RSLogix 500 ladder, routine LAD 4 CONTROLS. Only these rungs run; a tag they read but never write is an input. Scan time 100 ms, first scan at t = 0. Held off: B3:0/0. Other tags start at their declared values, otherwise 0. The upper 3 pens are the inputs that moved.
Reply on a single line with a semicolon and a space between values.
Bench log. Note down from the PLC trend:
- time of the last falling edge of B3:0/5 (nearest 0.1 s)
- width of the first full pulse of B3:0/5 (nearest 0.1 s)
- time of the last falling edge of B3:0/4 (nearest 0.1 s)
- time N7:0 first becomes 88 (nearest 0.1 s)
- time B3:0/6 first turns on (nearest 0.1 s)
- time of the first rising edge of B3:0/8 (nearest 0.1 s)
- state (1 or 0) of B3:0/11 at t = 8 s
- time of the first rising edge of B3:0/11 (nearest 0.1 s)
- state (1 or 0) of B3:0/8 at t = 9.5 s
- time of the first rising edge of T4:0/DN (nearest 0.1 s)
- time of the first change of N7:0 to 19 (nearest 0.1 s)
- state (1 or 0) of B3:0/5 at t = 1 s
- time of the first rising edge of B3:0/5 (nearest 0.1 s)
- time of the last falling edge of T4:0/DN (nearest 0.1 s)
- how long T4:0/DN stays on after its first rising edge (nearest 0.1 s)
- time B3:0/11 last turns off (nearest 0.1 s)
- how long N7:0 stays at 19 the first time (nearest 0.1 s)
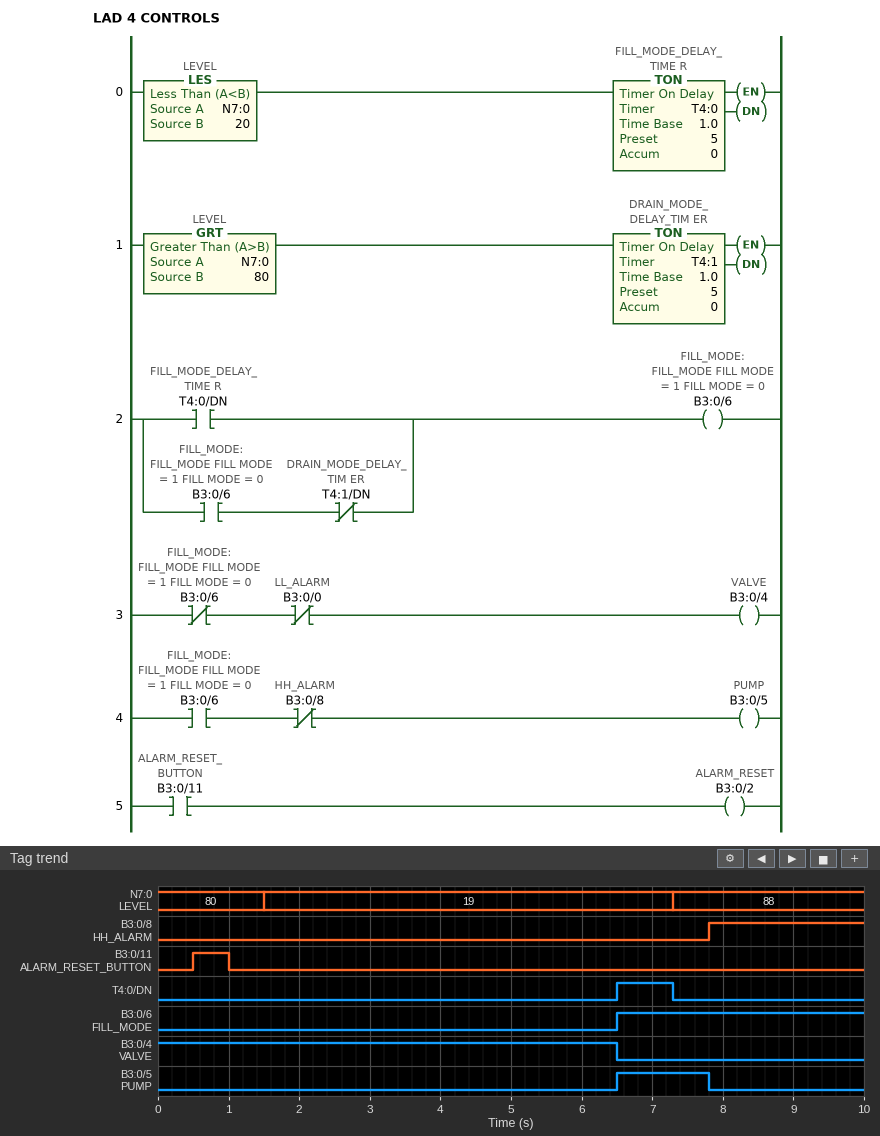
7.8 s; 1.3 s; 6.5 s; 7.3 s; 6.5 s; 7.8 s; 0; 0.5 s; 1; 6.5 s; 1.5 s; 0; 6.5 s; 7.3 s; 0.8 s; 1.0 s; 5.8 s
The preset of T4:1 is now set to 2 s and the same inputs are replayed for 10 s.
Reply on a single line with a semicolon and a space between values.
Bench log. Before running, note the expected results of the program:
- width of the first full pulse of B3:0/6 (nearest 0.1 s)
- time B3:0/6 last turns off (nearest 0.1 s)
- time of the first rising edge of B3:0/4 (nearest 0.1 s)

2.8 s; 9.3 s; 9.3 s
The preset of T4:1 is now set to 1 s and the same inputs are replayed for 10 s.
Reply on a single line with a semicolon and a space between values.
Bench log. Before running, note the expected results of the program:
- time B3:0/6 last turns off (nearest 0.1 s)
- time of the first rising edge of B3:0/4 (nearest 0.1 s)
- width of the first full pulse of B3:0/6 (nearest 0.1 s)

8.3 s; 8.3 s; 1.8 s
